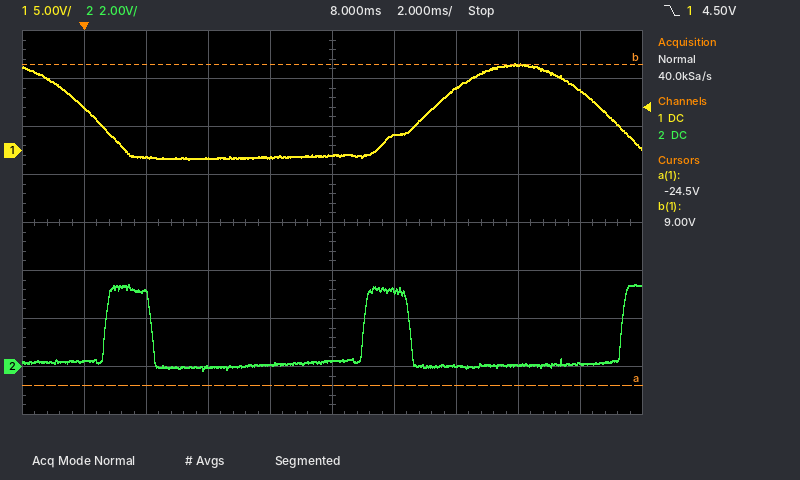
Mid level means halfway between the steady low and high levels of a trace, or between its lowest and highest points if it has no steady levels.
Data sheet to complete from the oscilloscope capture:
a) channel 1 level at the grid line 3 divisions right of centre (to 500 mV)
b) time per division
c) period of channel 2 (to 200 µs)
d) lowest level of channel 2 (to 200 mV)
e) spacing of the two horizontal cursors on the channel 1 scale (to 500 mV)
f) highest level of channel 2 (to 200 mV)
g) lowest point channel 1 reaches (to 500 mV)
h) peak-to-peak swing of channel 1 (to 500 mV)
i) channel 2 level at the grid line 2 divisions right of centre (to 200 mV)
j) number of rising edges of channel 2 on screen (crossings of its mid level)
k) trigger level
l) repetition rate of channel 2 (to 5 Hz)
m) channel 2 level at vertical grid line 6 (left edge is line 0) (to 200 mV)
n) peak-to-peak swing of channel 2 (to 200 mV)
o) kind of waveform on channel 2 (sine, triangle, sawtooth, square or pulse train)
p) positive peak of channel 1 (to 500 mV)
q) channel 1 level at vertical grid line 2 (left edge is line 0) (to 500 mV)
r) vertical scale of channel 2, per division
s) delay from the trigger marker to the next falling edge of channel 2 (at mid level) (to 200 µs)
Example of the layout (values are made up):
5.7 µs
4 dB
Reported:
9.0 V
2 ms
8.4 ms
-200 mV
33.5 V
3.4 V
-1.0 V
10.0 V
0.0 V
3
4.50 V
120 Hz
3.2 V
3.6 V
pulse train
9.0 V
-500 mV
2 V
2.2 ms
